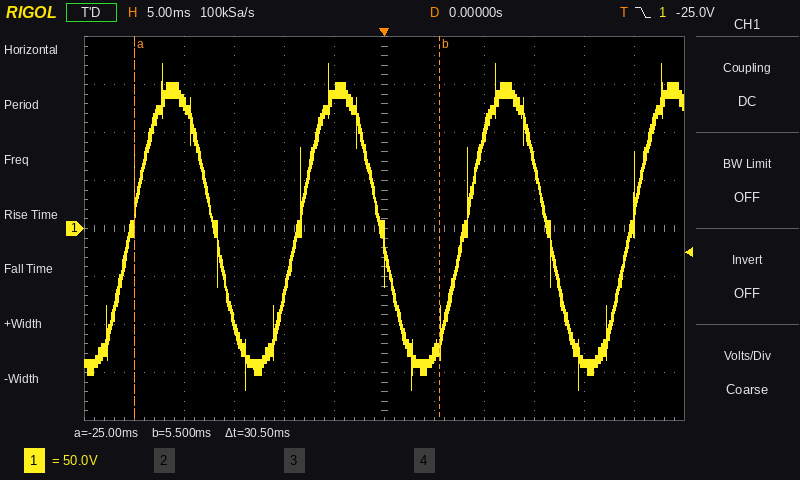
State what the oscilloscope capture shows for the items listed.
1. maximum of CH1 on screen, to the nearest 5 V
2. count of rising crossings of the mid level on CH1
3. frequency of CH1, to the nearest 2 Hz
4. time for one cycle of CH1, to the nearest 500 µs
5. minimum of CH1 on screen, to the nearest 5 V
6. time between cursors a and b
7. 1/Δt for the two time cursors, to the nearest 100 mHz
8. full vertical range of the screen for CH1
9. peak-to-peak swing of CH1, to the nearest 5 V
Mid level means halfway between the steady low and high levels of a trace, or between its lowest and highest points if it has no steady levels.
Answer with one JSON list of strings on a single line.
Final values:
["170 V", "4", "60 Hz", "16.5 ms", "-170 V", "30.5 ms", "32.8 Hz", "400 V", "340 V"]
